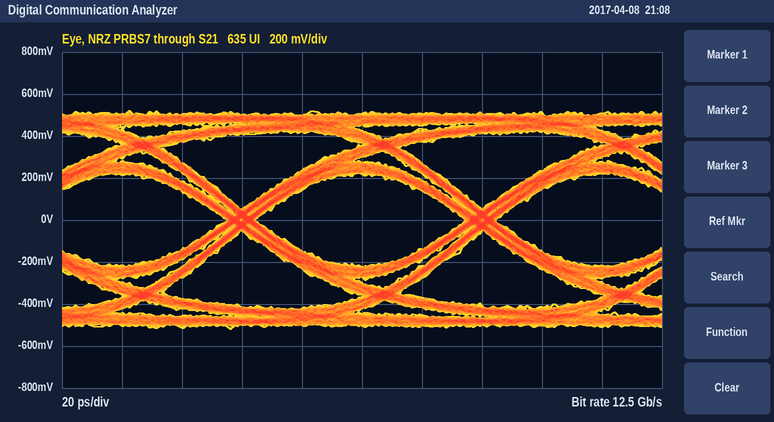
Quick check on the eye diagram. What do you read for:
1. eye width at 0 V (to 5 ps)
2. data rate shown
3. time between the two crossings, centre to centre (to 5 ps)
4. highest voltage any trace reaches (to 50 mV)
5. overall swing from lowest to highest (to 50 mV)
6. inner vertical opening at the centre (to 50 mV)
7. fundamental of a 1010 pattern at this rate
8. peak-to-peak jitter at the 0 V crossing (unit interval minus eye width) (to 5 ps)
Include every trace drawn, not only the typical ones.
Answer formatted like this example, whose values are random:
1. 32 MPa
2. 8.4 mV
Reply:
1. 70 ps
2. 12.5 Gb/s
3. 80 ps
4. 500 mV
5. 1.05 V
6. 450 mV
7. 6.25 GHz
8. 10 ps
